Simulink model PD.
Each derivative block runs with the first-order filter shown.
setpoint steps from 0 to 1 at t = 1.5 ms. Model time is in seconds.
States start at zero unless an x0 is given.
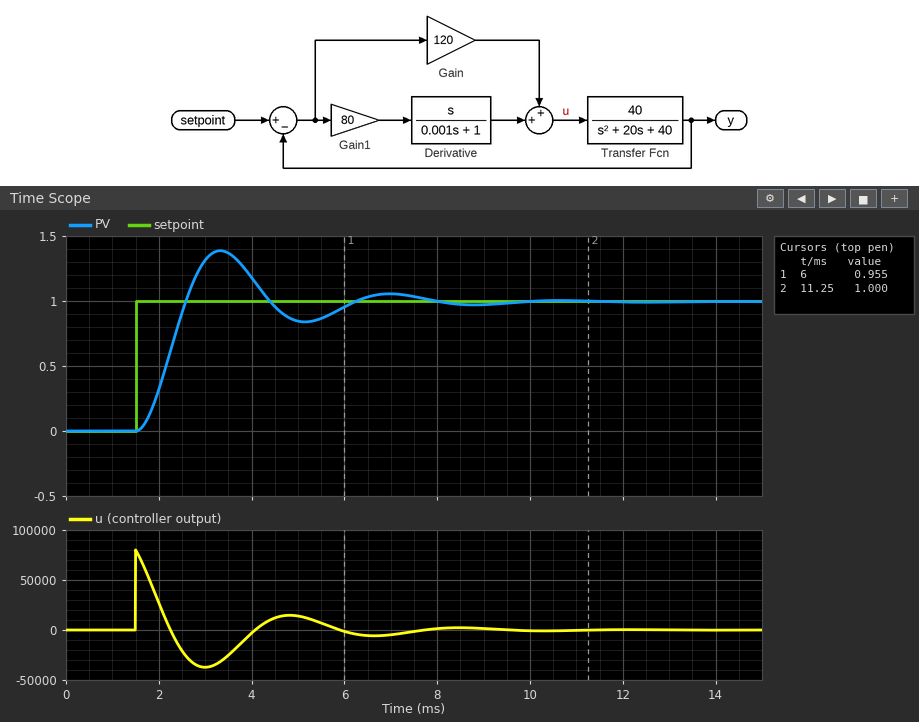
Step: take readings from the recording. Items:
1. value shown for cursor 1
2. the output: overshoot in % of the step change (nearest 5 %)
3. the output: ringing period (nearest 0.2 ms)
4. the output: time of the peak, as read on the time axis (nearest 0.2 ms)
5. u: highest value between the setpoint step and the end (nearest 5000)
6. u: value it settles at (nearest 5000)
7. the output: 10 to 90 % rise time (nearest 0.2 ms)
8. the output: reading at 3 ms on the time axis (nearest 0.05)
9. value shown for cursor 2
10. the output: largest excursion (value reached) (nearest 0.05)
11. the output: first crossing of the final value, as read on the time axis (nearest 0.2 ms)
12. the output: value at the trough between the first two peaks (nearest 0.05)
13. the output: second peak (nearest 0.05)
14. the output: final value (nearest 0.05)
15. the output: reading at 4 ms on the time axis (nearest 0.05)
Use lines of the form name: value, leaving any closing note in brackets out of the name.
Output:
value shown for cursor 1: 0.955
the output: overshoot in % of the step change: 40 %
the output: ringing period: 3.6 ms
the output: time of the peak, as read on the time axis: 3.4 ms
u: highest value between the setpoint step and the end: 80000
u: value it settles at: 0
the output: 10 to 90 % rise time: 0.8 ms
the output: reading at 3 ms on the time axis: 1.30
value shown for cursor 2: 1.000
the output: largest excursion (value reached): 1.40
the output: first crossing of the final value, as read on the time axis: 2.6 ms
the output: value at the trough between the first two peaks: 0.85
the output: second peak: 1.05
the output: final value: 1.00
the output: reading at 4 ms on the time axis: 1.20
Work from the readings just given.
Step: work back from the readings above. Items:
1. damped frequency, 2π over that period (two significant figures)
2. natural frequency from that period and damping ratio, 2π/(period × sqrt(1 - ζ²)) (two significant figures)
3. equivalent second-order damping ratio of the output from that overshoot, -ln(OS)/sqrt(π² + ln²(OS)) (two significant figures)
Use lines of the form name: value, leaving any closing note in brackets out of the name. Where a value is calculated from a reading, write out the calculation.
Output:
damped frequency, 2π over that period: 2π / 3.6 = 1.7 rad/ms
natural frequency from that period and damping ratio, 2π/(period × sqrt(1 - ζ²)): 2π / (3.6 × sqrt(1 - 0.28²)) = 1.8 rad/ms
equivalent second-order damping ratio of the output from that overshoot, -ln(OS)/sqrt(π² + ln²(OS)): ln(0.4) = -0.916; 0.916 / sqrt(9.870 + 0.840) = 0.28
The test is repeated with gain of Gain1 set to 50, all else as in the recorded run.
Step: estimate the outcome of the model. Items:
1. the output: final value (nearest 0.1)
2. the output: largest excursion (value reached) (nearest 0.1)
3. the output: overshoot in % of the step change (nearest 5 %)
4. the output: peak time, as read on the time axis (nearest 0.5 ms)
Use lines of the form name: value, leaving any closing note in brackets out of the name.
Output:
the output: final value: 1.0
the output: largest excursion (value reached): 1.3
the output: overshoot in % of the step change: 30 %
the output: peak time, as read on the time axis: 4.0 ms
